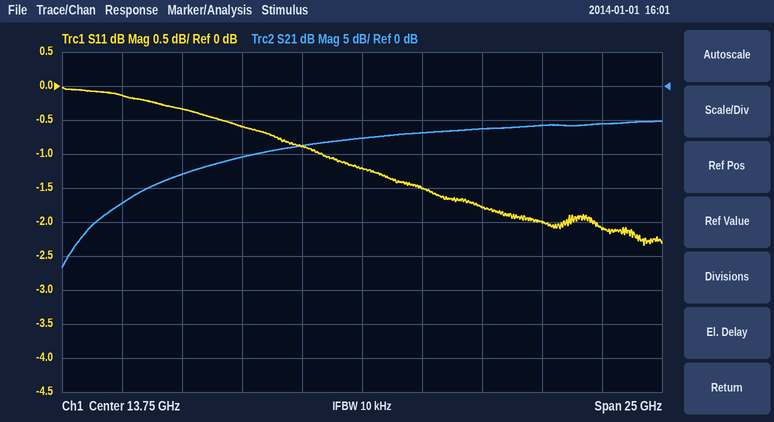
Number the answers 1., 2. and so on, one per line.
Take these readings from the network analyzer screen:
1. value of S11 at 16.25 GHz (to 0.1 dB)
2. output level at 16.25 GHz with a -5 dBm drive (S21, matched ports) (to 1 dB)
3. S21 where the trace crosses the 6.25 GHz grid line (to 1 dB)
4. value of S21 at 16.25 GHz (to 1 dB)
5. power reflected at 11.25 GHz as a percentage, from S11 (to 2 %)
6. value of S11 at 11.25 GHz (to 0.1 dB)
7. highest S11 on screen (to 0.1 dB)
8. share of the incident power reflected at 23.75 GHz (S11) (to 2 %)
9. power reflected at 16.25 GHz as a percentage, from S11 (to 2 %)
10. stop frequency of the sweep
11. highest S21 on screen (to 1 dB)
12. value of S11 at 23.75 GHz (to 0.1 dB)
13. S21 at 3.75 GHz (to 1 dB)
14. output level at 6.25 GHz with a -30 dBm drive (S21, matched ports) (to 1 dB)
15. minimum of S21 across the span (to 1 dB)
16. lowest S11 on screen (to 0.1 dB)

1. -1.5 dB
2. -12 dBm
3. -13 dB
4. -7 dB
5. 82 %
6. -0.9 dB
7. 0.0 dB
8. 62 %
9. 70 %
10. 26.25 GHz
11. -5 dB
12. -2.1 dB
13. -17 dB
14. -43 dBm
15. -27 dB
16. -2.3 dB
